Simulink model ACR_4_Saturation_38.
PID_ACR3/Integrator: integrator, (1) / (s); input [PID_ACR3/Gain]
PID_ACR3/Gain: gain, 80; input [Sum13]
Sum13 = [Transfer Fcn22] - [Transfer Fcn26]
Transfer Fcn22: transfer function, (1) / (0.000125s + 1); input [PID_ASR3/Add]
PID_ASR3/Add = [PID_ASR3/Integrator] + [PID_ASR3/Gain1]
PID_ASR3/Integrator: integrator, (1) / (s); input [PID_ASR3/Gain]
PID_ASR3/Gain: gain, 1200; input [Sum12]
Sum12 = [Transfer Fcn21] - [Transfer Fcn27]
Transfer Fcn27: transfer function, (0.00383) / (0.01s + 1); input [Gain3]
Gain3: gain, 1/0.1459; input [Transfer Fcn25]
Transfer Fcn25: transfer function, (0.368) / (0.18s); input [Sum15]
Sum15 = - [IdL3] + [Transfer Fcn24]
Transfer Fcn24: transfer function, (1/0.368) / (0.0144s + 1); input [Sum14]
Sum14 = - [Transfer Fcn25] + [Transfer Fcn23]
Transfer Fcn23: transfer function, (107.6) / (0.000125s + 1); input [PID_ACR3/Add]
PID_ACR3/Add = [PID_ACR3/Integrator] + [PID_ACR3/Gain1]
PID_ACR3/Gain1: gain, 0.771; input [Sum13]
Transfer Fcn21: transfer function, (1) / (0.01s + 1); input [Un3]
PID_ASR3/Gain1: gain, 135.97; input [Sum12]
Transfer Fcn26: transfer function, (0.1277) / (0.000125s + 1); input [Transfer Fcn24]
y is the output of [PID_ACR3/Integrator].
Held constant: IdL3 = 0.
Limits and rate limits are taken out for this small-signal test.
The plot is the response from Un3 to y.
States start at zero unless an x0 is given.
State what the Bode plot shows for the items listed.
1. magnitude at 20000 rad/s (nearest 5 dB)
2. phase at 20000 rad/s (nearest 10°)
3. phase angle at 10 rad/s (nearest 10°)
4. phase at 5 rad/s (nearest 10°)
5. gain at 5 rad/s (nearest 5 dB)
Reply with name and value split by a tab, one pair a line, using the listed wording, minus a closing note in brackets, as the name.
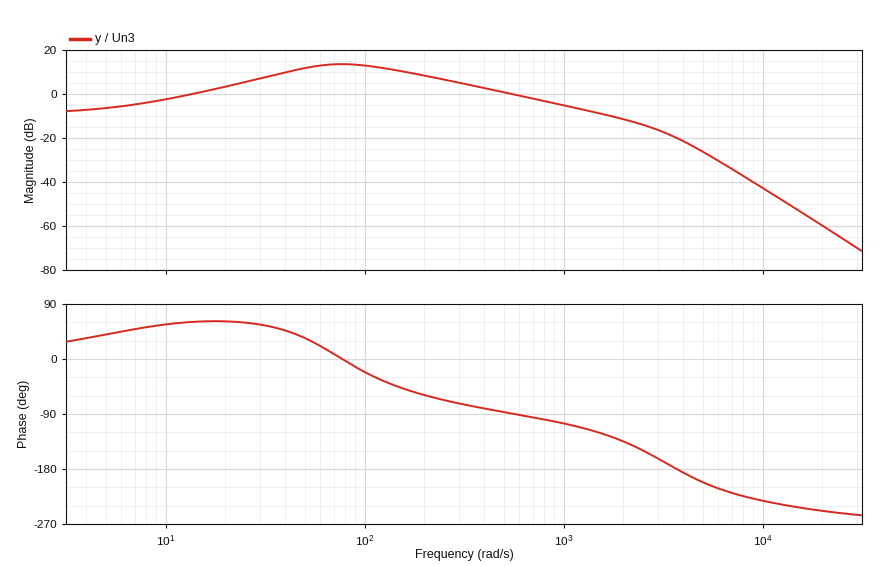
magnitude at 20000 rad/s	-60 dB
phase at 20000 rad/s	-250°
phase angle at 10 rad/s	60°
phase at 5 rad/s	40°
gain at 5 rad/s	-5 dB
